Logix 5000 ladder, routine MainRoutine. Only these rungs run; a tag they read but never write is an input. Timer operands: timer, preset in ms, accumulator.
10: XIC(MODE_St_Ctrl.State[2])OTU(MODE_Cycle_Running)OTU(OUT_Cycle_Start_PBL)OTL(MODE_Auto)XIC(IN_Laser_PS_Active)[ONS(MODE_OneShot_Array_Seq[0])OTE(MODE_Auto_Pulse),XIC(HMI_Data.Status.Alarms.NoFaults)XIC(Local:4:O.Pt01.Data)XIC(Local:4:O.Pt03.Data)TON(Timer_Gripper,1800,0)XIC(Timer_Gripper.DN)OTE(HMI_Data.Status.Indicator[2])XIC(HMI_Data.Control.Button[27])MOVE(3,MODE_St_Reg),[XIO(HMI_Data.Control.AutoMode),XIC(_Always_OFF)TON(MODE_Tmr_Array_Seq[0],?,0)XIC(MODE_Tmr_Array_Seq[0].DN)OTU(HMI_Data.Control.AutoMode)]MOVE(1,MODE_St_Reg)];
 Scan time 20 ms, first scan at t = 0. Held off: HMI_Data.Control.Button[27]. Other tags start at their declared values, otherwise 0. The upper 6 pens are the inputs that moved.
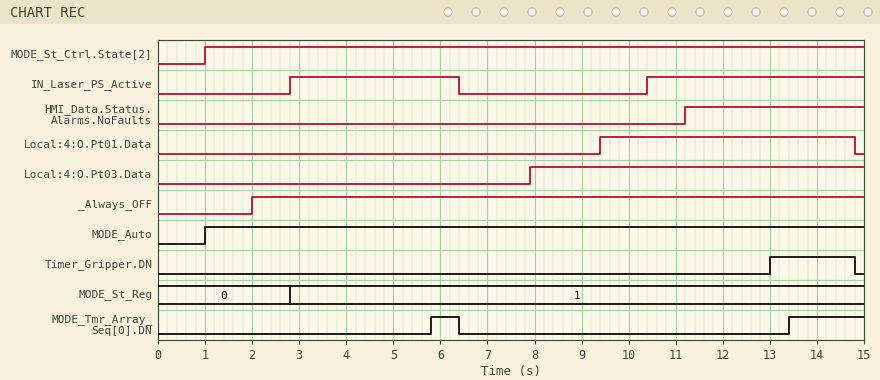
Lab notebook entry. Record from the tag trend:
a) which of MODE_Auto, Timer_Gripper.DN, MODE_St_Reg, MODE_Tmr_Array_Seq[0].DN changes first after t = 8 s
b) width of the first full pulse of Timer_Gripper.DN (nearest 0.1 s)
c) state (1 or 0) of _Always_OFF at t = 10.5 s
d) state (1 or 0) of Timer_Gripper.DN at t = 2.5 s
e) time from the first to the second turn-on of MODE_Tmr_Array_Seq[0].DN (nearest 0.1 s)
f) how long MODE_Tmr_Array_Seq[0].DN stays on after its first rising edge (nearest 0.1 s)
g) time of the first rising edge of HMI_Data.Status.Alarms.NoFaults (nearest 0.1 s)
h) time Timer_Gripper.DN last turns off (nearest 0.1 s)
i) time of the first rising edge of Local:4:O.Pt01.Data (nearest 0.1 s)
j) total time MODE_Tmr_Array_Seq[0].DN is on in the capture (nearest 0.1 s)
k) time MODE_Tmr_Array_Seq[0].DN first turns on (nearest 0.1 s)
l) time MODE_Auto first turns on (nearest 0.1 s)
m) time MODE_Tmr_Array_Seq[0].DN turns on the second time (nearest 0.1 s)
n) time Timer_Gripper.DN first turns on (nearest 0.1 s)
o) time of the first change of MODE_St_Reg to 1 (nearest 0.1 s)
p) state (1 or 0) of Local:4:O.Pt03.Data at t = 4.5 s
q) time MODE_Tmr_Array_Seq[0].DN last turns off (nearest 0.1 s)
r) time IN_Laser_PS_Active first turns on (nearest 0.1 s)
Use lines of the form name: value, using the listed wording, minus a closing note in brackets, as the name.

which of MODE_Auto, Timer_Gripper.DN, MODE_St_Reg, MODE_Tmr_Array_Seq[0].DN changes first after t = 8 s: Timer_Gripper.DN
width of the first full pulse of Timer_Gripper.DN: 1.8 s
state (1 or 0) of _Always_OFF at t = 10.5 s: 1
state (1 or 0) of Timer_Gripper.DN at t = 2.5 s: 0
time from the first to the second turn-on of MODE_Tmr_Array_Seq[0].DN: 7.6 s
how long MODE_Tmr_Array_Seq[0].DN stays on after its first rising edge: 0.6 s
time of the first rising edge of HMI_Data.Status.Alarms.NoFaults: 11.2 s
time Timer_Gripper.DN last turns off: 14.8 s
time of the first rising edge of Local:4:O.Pt01.Data: 9.4 s
total time MODE_Tmr_Array_Seq[0].DN is on in the capture: 2.2 s
time MODE_Tmr_Array_Seq[0].DN first turns on: 5.8 s
time MODE_Auto first turns on: 1.0 s
time MODE_Tmr_Array_Seq[0].DN turns on the second time: 13.4 s
time Timer_Gripper.DN first turns on: 13.0 s
time of the first change of MODE_St_Reg to 1: 2.8 s
state (1 or 0) of Local:4:O.Pt03.Data at t = 4.5 s: 0
time MODE_Tmr_Array_Seq[0].DN last turns off: 6.4 s
time IN_Laser_PS_Active first turns on: 2.8 s
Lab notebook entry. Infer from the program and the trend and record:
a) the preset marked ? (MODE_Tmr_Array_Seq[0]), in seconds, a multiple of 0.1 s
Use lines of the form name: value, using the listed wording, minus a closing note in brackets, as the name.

the preset marked ? (MODE_Tmr_Array_Seq[0]), in seconds, a multiple of 0.1 s: 3.0 s
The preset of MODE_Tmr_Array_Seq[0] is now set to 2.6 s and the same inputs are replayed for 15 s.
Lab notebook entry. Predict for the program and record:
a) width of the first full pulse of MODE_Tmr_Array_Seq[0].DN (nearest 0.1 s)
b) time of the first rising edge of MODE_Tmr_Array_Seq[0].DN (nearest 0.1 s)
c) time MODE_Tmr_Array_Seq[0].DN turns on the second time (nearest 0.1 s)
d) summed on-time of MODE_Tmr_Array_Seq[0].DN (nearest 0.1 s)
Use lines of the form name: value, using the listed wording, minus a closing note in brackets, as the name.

width of the first full pulse of MODE_Tmr_Array_Seq[0].DN: 1.0 s
time of the first rising edge of MODE_Tmr_Array_Seq[0].DN: 5.4 s
time MODE_Tmr_Array_Seq[0].DN turns on the second time: 13.0 s
summed on-time of MODE_Tmr_Array_Seq[0].DN: 3.0 s
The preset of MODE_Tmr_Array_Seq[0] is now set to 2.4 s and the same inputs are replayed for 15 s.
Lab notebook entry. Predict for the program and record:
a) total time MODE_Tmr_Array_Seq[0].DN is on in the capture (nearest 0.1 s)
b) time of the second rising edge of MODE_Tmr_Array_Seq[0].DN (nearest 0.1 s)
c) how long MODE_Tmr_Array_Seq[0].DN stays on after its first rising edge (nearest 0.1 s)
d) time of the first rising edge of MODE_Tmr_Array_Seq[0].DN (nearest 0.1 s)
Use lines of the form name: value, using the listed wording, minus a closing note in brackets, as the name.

total time MODE_Tmr_Array_Seq[0].DN is on in the capture: 3.4 s
time of the second rising edge of MODE_Tmr_Array_Seq[0].DN: 12.8 s
how long MODE_Tmr_Array_Seq[0].DN stays on after its first rising edge: 1.2 s
time of the first rising edge of MODE_Tmr_Array_Seq[0].DN: 5.2 s
